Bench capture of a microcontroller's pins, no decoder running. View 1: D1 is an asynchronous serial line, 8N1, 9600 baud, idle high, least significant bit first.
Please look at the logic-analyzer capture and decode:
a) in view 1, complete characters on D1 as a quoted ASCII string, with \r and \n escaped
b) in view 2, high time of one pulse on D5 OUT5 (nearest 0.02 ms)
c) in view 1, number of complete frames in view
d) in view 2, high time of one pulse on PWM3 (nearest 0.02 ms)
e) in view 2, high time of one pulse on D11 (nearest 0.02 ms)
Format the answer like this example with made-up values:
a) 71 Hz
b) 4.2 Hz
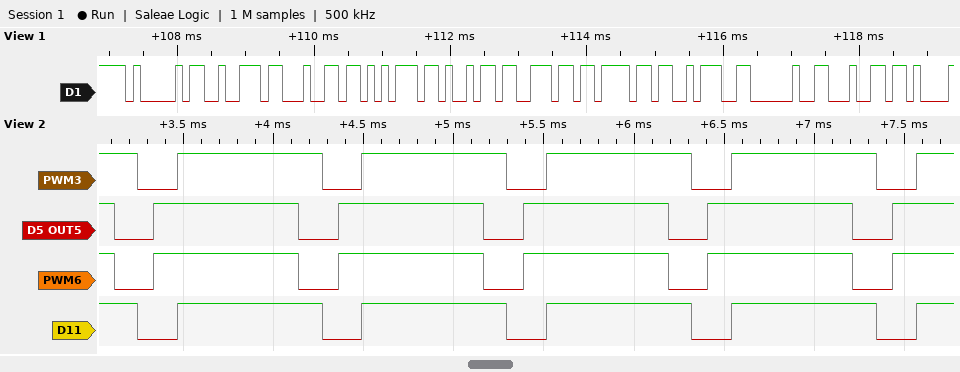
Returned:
a) "Arduino: d"
b) 0.80 ms
c) 10
d) 0.80 ms
e) 0.80 ms
